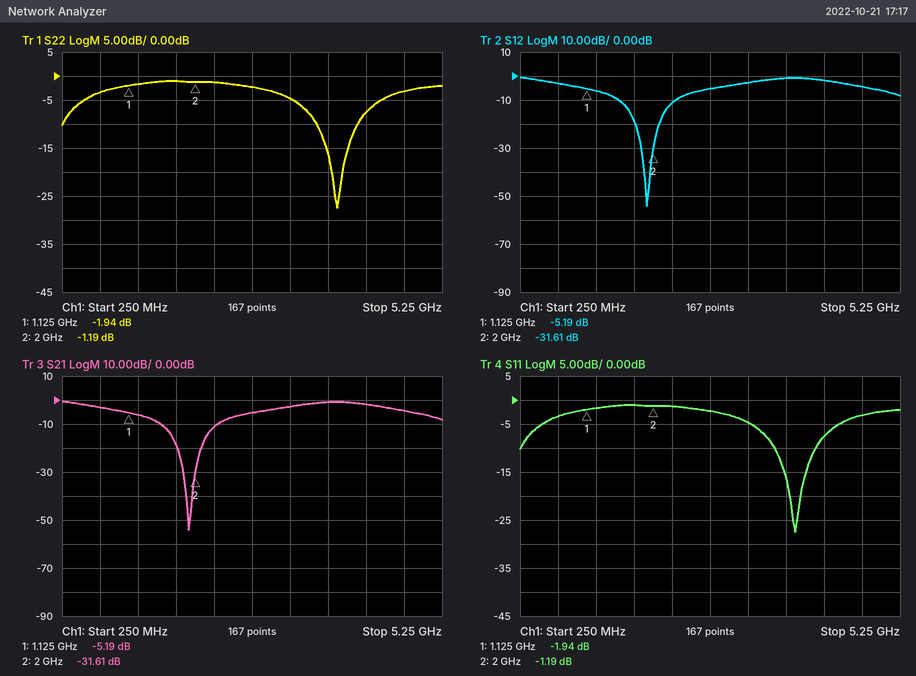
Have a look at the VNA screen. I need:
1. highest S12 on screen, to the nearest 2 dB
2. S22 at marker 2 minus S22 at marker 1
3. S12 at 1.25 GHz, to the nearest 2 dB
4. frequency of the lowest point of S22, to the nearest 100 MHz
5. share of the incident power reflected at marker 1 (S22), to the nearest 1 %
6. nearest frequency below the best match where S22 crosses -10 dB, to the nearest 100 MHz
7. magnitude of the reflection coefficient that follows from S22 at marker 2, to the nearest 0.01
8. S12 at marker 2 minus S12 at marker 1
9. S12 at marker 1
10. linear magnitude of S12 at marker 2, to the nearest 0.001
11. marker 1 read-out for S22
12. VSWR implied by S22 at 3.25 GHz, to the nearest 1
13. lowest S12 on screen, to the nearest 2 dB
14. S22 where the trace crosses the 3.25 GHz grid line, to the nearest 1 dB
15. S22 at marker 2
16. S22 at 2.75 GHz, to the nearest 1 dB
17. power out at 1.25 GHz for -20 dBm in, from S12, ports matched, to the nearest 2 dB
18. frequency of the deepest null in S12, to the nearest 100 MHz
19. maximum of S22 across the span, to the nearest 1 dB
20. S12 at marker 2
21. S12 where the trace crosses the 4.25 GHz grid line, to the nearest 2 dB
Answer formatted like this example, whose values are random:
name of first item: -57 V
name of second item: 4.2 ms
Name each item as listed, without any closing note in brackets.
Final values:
highest S12 on screen, to the nearest 2 dB: 0 dB
S22 at marker 2 minus S22 at marker 1: 0.75 dB
S12 at 1.25 GHz, to the nearest 2 dB: -6 dB
frequency of the lowest point of S22, to the nearest 100 MHz: 3.9 GHz
share of the incident power reflected at marker 1 (S22), to the nearest 1 %: 64 %
nearest frequency below the best match where S22 crosses -10 dB, to the nearest 100 MHz: 3.6 GHz
magnitude of the reflection coefficient that follows from S22 at marker 2, to the nearest 0.01: 0.87
S12 at marker 2 minus S12 at marker 1: -26.42 dB
S12 at marker 1: -5.19 dB
linear magnitude of S12 at marker 2, to the nearest 0.001: 0.026
marker 1 read-out for S22: -1.94 dB
VSWR implied by S22 at 3.25 GHz, to the nearest 1: 4
lowest S12 on screen, to the nearest 2 dB: -54 dB
S22 where the trace crosses the 3.25 GHz grid line, to the nearest 1 dB: -5 dB
S22 at marker 2: -1.19 dB
S22 at 2.75 GHz, to the nearest 1 dB: -2 dB
power out at 1.25 GHz for -20 dBm in, from S12, ports matched, to the nearest 2 dB: -26 dBm
frequency of the deepest null in S12, to the nearest 100 MHz: 1.9 GHz
maximum of S22 across the span, to the nearest 1 dB: -1 dB
S12 at marker 2: -31.61 dB
S12 where the trace crosses the 4.25 GHz grid line, to the nearest 2 dB: -2 dB
